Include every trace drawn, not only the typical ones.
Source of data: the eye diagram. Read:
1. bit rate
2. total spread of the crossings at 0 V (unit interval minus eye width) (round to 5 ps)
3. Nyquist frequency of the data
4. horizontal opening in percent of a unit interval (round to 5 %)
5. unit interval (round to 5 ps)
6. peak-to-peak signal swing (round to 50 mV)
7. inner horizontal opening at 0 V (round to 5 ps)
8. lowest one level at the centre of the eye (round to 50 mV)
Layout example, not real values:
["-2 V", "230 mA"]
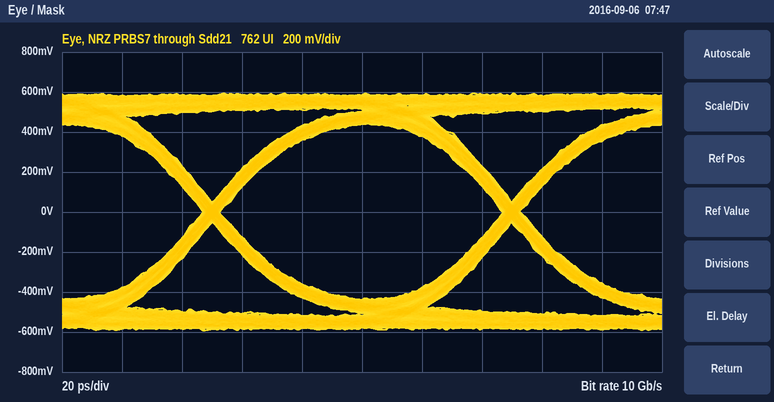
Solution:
["10 Gb/s", "5 ps", "5 GHz", "95 %", "100 ps", "1.20 V", "95 ps", "450 mV"]
